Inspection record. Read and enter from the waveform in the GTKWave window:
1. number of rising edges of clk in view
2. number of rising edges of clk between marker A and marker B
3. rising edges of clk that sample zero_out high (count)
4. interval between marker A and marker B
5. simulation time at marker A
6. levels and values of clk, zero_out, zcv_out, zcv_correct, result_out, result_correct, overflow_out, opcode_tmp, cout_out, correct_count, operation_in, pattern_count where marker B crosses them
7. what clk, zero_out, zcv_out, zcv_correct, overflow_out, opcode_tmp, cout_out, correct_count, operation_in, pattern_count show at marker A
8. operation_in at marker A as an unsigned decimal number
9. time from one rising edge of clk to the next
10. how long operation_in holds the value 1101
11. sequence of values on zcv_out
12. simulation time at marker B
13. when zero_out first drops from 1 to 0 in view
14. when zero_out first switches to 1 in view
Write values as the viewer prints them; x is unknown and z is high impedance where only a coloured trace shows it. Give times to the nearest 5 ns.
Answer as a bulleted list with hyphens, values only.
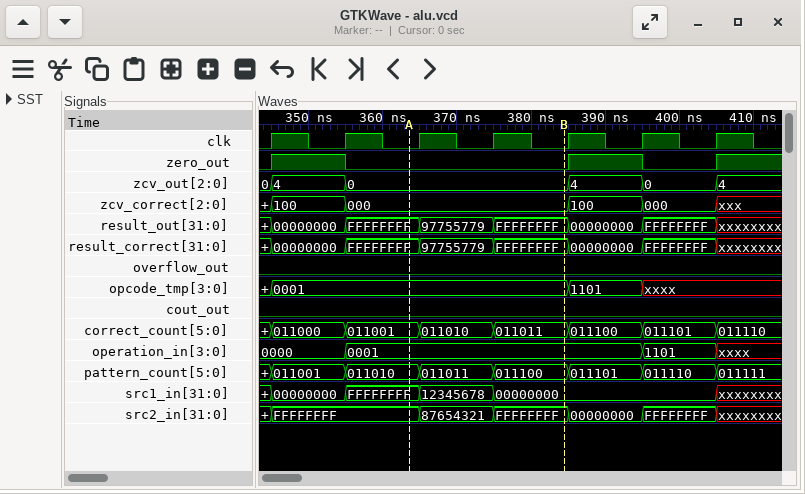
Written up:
- 7
- 2
- 2
- 20 ns
- 365 ns
- clk=0, zero_out=0, zcv_out=0, zcv_correct=000, result_out=FFFFFFFF, result_correct=FFFFFFFF, overflow_out=0, opcode_tmp=0001, cout_out=0, correct_count=011011, operation_in=0001, pattern_count=011100
- clk=0, zero_out=0, zcv_out=0, zcv_correct=000, overflow_out=0, opcode_tmp=0001, cout_out=0, correct_count=011001, operation_in=0001, pattern_count=011010
- 1
- 10 ns
- 10 ns
- 0, 4, 0, 4, 0, 4
- 385 ns
- 355 ns
- 345 ns
